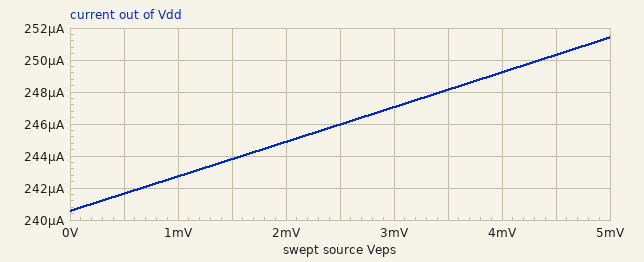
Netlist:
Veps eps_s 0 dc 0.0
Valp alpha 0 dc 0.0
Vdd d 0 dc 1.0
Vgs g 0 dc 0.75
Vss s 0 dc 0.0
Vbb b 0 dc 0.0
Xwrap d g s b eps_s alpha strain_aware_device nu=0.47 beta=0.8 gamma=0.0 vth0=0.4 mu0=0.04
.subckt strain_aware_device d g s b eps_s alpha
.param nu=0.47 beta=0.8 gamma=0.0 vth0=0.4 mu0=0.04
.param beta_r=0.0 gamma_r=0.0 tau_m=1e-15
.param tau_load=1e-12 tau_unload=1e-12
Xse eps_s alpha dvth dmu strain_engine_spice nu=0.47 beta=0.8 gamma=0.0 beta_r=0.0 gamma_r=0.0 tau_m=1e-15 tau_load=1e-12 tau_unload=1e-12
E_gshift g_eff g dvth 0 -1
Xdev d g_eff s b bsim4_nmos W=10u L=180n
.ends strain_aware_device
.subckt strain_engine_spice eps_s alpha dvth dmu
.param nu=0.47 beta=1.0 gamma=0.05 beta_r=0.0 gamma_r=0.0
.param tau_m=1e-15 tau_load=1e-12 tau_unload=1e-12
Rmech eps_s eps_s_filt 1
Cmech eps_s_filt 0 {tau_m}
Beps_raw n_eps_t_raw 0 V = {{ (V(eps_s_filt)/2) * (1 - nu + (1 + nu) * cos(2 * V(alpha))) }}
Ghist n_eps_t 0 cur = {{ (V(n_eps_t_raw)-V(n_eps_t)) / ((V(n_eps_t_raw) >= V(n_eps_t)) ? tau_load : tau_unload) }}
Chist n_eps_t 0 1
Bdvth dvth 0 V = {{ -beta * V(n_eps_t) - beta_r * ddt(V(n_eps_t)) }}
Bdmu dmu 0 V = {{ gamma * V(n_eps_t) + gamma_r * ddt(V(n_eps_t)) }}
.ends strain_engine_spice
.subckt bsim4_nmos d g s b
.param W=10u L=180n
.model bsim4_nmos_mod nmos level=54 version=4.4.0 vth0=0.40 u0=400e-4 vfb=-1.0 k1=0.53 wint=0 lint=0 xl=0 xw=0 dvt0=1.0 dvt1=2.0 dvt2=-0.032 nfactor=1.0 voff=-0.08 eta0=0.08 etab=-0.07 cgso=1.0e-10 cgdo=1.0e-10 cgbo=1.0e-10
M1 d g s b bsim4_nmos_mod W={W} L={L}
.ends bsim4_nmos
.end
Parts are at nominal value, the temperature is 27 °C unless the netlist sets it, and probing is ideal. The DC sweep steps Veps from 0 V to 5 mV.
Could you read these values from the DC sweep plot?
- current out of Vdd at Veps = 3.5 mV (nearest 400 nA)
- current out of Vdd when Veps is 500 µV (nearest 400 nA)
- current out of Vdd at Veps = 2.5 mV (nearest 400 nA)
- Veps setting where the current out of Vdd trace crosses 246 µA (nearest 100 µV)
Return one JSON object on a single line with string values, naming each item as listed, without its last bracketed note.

{"current out of Vdd at Veps = 3.5 mV": "248.0 µA", "current out of Vdd when Veps is 500 µV": "241.6 µA", "current out of Vdd at Veps = 2.5 mV": "246.0 µA", "Veps setting where the current out of Vdd trace crosses 246 µA": "2.5 mV"}
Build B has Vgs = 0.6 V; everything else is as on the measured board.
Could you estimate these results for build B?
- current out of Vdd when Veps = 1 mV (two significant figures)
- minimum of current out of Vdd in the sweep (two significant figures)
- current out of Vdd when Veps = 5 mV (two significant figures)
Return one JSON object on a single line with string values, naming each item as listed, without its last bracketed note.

{"current out of Vdd when Veps = 1 mV": "16 µA", "minimum of current out of Vdd in the sweep": "15 µA", "current out of Vdd when Veps = 5 mV": "17 µA"}
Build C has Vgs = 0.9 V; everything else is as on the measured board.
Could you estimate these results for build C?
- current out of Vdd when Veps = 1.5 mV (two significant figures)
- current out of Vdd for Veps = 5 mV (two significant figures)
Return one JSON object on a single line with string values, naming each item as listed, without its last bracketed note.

{"current out of Vdd when Veps = 1.5 mV": "740 µA", "current out of Vdd for Veps = 5 mV": "750 µA"}
